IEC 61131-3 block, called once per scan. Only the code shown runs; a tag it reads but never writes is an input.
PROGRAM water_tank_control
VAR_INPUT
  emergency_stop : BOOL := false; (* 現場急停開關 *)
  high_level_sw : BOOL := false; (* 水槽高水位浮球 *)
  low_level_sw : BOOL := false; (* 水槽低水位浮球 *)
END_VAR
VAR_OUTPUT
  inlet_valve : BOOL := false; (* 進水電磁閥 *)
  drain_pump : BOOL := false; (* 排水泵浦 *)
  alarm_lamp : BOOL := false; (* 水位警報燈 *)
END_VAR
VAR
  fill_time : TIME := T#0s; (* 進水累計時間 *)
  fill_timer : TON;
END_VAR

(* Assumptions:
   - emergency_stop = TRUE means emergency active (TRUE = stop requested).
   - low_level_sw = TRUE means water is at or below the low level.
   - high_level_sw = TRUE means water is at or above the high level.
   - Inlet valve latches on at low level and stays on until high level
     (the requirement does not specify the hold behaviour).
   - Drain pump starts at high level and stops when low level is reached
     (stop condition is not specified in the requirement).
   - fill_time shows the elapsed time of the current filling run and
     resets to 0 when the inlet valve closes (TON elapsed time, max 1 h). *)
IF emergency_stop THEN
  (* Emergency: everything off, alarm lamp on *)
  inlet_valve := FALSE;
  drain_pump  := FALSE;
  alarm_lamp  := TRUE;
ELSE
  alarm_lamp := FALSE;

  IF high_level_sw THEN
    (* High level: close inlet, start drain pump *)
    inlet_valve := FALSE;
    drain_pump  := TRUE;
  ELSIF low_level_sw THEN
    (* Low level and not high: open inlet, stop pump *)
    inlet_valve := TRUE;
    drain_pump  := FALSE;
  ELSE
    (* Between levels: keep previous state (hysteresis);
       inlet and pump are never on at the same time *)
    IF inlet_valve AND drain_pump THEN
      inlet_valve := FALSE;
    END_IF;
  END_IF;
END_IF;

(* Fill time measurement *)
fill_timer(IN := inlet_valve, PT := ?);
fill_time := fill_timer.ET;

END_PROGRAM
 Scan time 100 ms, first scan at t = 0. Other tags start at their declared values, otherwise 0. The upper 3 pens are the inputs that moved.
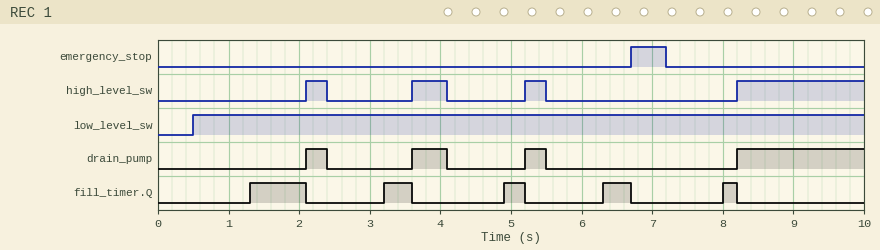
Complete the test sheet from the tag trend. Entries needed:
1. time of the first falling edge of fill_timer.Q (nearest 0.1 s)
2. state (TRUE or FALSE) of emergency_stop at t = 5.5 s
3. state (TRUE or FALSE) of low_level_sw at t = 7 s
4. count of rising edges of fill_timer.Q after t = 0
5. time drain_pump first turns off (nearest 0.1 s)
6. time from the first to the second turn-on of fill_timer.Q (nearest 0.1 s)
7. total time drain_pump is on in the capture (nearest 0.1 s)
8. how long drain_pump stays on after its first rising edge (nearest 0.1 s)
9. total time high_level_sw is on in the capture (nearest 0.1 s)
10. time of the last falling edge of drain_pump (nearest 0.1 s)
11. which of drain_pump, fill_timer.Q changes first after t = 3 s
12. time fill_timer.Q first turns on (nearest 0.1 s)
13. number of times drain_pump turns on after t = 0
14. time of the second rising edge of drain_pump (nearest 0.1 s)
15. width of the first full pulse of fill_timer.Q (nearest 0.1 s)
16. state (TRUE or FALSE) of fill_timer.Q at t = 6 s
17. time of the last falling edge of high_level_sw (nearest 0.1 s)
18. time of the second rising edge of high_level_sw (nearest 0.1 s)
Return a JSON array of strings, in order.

["2.1 s", "FALSE", "TRUE", "5", "2.4 s", "1.9 s", "2.9 s", "0.3 s", "2.9 s", "5.5 s", "fill_timer.Q", "1.3 s", "4", "3.6 s", "0.8 s", "FALSE", "5.5 s", "3.6 s"]
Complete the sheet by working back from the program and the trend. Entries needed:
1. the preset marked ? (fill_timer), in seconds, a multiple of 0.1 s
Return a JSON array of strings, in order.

["0.8 s"]
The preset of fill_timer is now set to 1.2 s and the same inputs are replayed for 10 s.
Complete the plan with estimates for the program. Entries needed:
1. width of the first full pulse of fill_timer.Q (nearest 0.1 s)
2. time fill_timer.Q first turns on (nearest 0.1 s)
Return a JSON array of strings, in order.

["0.4 s", "1.7 s"]
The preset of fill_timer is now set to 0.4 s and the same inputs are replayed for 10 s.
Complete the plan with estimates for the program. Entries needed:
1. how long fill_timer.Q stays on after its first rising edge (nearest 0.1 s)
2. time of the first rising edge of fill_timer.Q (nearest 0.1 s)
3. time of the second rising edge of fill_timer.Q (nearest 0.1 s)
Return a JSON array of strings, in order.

["1.2 s", "0.9 s", "2.8 s"]
